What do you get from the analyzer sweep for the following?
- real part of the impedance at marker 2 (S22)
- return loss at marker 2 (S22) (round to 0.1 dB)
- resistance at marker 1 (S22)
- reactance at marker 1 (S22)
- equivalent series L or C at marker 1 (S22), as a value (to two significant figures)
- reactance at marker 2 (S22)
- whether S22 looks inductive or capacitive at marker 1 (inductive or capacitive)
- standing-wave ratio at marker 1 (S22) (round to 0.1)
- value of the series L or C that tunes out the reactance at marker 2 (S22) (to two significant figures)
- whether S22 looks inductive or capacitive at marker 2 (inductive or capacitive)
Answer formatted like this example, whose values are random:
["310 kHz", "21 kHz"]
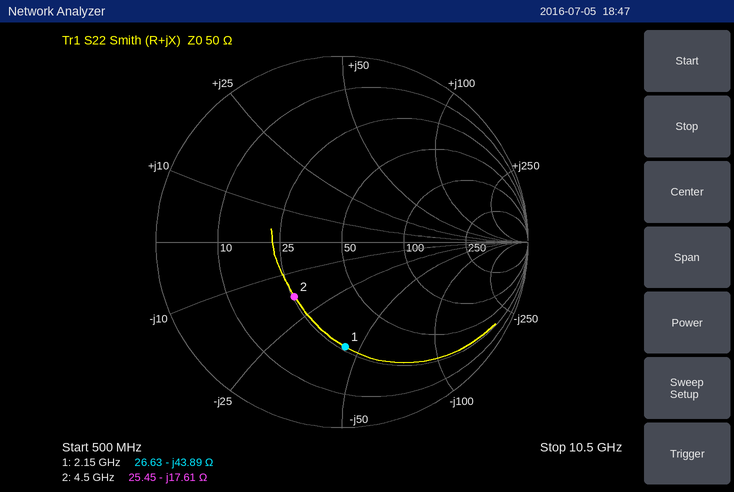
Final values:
["25.45 Ω", "8.2 dB", "26.63 Ω", "-43.89 Ω", "1.7 pF", "-17.61 Ω", "capacitive", "3.6", "620 pH", "capacitive"]
